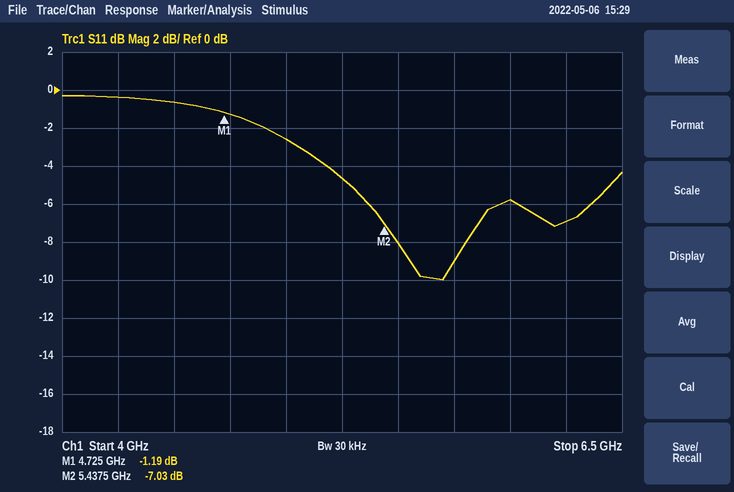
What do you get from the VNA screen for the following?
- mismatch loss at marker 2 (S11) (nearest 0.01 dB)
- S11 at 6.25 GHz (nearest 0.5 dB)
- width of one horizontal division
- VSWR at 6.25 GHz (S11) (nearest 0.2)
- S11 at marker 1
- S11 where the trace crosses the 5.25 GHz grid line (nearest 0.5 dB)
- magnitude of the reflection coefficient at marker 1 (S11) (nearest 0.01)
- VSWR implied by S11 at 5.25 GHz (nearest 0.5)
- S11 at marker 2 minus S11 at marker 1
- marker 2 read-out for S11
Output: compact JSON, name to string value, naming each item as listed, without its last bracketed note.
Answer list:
{"mismatch loss at marker 2 (S11)": "0.96 dB", "S11 at 6.25 GHz": "-7.0 dB", "width of one horizontal division": "250 MHz", "VSWR at 6.25 GHz (S11)": "2.6", "S11 at marker 1": "-1.19 dB", "S11 where the trace crosses the 5.25 GHz grid line": "-4.5 dB", "magnitude of the reflection coefficient at marker 1 (S11)": "0.87", "VSWR implied by S11 at 5.25 GHz": "4.0", "S11 at marker 2 minus S11 at marker 1": "-5.84 dB", "marker 2 read-out for S11": "-7.03 dB"}
